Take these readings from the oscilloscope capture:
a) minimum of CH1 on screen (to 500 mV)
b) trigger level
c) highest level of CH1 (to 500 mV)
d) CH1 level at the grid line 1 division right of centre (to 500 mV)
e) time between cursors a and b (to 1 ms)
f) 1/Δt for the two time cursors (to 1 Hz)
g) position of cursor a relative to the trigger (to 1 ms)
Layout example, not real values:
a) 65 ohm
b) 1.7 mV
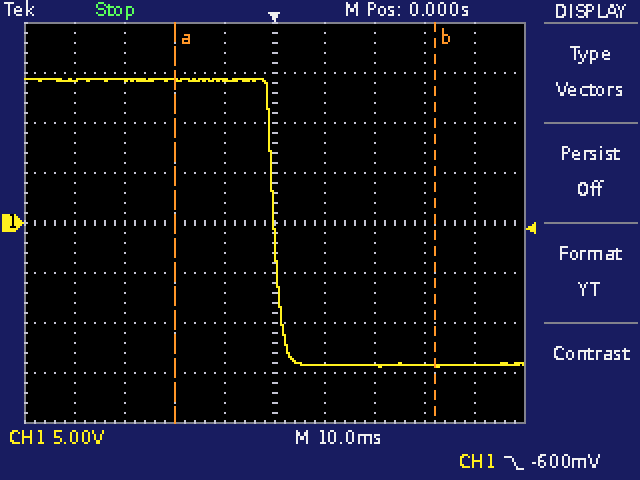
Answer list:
a) -14.5 V
b) -600 mV
c) 14.5 V
d) -14.0 V
e) 52 ms
f) 19 Hz
g) -20 ms
